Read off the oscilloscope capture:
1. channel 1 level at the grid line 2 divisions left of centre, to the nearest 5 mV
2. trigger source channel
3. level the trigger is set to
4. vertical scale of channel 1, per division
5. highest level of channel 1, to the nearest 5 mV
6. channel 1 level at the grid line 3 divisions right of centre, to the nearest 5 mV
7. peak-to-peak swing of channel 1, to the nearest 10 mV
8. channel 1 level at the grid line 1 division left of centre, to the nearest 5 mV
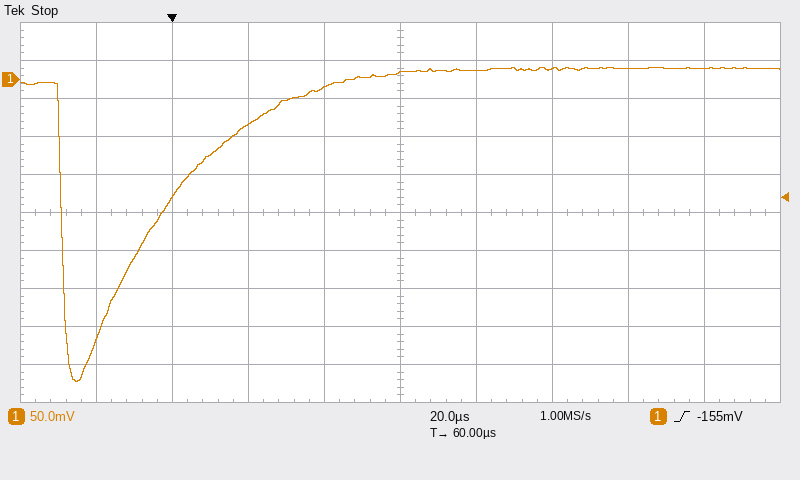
-60 mV
channel 1
-155 mV
50 mV
15 mV
15 mV
410 mV
-10 mV
